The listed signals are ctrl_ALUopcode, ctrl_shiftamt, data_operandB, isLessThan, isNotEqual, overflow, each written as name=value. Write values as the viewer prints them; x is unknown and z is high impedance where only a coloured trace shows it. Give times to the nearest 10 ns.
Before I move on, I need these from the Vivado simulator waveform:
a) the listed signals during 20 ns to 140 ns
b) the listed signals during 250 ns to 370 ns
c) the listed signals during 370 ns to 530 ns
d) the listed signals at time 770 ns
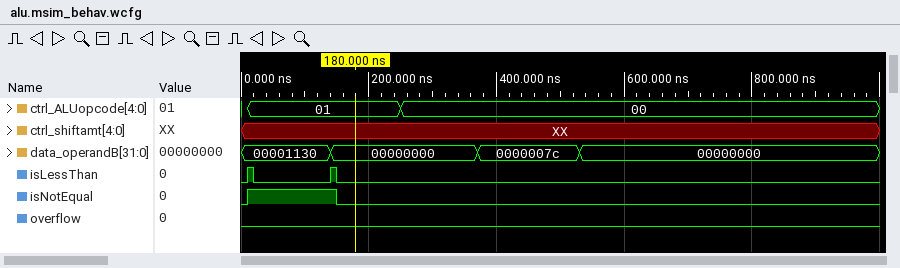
ctrl_ALUopcode=01, ctrl_shiftamt=XX, data_operandB=00001130, isLessThan=0, isNotEqual=1, overflow=0
ctrl_ALUopcode=00, ctrl_shiftamt=XX, data_operandB=00000000, isLessThan=0, isNotEqual=0, overflow=0
ctrl_ALUopcode=00, ctrl_shiftamt=XX, data_operandB=0000007c, isLessThan=0, isNotEqual=0, overflow=0
ctrl_ALUopcode=00, ctrl_shiftamt=XX, data_operandB=00000000, isLessThan=0, isNotEqual=0, overflow=0
